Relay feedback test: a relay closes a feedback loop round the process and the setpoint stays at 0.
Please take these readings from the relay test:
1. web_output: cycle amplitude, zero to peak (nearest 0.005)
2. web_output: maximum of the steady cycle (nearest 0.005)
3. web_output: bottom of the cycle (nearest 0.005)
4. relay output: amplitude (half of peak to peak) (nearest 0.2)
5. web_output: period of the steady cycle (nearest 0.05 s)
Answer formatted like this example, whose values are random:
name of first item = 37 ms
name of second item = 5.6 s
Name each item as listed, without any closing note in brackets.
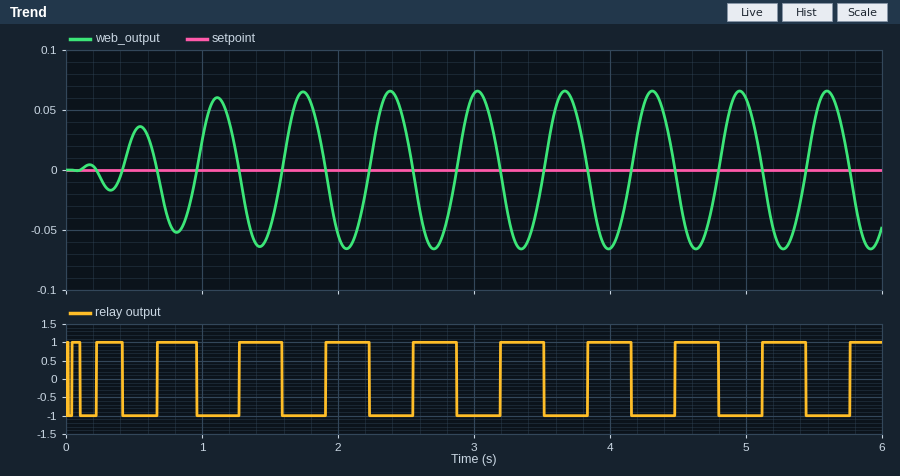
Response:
web_output: cycle amplitude, zero to peak = 0.065
web_output: maximum of the steady cycle = 0.065
web_output: bottom of the cycle = -0.065
relay output: amplitude (half of peak to peak) = 1.0
web_output: period of the steady cycle = 0.65 s
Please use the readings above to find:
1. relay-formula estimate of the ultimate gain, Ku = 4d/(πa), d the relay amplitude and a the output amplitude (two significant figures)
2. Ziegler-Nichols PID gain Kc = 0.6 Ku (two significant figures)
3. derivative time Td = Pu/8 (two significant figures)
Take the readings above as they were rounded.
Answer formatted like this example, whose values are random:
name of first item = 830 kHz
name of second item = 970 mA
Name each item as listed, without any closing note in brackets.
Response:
relay-formula estimate of the ultimate gain, Ku = 4d/(πa), d the relay amplitude and a the output amplitude = 20
Ziegler-Nichols PID gain Kc = 0.6 Ku = 12
derivative time Td = Pu/8 = 0.081 s
